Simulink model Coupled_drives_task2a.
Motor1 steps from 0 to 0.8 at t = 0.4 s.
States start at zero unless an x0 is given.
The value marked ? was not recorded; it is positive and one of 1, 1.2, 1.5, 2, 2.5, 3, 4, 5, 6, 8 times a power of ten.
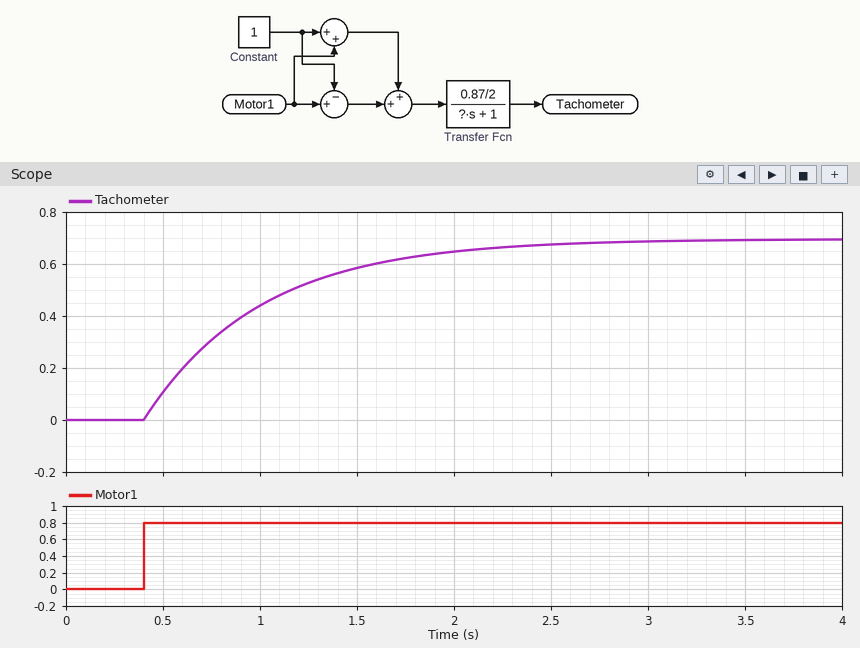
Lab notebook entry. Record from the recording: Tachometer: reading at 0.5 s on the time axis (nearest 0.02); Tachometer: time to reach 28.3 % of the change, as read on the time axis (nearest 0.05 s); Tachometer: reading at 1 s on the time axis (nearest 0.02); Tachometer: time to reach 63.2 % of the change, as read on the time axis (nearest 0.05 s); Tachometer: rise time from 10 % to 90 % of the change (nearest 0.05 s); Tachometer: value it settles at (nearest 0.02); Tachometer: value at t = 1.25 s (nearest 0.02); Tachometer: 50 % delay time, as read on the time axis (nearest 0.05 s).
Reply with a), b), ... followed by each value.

a) 0.10
b) 0.60 s
c) 0.44
d) 1.00 s
e) 1.30 s
f) 0.70
g) 0.52
h) 0.80 s
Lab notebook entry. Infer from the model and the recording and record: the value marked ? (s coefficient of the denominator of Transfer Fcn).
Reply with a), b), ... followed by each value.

a) 0.6
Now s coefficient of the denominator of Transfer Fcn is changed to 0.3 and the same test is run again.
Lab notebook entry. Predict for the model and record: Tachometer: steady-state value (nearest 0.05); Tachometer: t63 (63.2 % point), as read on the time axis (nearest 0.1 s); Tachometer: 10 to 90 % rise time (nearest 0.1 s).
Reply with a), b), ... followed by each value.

a) 0.70
b) 0.7 s
c) 0.7 s
